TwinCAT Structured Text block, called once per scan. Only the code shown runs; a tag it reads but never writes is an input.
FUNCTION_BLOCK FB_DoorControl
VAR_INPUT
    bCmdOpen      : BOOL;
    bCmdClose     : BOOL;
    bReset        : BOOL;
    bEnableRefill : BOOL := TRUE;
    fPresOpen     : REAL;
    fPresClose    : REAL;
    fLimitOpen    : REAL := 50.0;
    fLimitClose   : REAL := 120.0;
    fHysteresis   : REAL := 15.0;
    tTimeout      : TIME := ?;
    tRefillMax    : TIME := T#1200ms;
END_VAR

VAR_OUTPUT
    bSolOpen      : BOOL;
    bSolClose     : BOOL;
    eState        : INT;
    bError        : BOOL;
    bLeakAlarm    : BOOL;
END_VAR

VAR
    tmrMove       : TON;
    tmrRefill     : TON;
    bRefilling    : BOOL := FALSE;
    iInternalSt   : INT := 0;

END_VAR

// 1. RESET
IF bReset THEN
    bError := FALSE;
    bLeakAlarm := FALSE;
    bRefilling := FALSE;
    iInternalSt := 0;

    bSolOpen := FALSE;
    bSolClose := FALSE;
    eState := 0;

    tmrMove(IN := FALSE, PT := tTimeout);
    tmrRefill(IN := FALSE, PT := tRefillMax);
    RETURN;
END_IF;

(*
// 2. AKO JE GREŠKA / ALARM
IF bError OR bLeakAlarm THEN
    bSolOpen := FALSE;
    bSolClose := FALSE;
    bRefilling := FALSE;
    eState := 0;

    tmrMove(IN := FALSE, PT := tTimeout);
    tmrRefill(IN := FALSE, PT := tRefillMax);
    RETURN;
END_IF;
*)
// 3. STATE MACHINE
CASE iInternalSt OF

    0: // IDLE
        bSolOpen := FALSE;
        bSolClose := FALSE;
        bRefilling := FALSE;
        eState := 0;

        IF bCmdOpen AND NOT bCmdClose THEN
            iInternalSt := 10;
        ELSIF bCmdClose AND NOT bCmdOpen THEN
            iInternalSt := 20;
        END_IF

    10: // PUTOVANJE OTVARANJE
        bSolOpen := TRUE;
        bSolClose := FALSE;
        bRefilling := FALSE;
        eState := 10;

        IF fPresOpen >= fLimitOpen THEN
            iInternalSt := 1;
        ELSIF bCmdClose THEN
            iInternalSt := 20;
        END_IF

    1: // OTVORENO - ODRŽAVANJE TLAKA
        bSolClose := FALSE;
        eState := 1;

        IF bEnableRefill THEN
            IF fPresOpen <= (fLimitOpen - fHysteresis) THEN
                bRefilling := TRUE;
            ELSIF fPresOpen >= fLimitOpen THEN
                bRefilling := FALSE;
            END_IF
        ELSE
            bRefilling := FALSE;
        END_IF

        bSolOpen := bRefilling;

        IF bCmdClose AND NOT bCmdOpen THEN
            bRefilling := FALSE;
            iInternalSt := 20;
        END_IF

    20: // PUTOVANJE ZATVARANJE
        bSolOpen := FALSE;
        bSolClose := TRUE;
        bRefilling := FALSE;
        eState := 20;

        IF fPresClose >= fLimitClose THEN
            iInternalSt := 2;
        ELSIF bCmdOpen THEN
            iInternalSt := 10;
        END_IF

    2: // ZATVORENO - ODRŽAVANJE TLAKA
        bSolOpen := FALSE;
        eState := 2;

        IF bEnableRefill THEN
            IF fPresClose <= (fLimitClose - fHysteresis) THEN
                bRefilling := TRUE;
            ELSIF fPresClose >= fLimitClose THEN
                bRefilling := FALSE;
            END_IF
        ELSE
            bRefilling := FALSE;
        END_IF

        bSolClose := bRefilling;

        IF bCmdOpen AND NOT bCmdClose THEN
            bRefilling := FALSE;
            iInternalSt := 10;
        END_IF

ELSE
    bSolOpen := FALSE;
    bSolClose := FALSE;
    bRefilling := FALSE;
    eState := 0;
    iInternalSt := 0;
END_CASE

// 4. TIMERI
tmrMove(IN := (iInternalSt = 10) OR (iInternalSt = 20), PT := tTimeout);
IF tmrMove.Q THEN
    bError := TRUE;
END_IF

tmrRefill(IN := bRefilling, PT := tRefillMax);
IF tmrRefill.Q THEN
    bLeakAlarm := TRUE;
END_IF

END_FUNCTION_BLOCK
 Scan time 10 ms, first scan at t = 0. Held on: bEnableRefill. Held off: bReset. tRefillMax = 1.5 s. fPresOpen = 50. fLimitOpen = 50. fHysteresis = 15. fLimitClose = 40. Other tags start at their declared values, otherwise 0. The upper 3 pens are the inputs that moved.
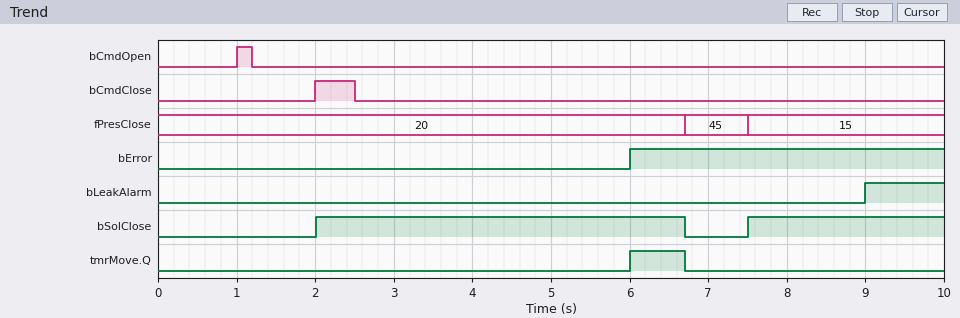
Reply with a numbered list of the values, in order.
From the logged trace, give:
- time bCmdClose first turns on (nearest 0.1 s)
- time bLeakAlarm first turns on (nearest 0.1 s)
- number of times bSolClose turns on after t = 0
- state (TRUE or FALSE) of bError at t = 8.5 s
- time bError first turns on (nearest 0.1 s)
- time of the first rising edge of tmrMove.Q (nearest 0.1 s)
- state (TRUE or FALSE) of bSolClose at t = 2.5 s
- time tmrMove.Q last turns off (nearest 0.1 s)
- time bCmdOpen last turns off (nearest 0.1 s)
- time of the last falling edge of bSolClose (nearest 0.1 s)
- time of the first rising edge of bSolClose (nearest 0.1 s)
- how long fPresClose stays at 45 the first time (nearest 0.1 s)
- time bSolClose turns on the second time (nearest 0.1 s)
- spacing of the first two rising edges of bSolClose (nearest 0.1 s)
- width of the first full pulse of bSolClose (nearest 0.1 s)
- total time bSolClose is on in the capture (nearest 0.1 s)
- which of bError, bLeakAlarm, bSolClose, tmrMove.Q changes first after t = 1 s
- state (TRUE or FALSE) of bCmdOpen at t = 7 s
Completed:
1. 2.0 s
2. 9.0 s
3. 2
4. TRUE
5. 6.0 s
6. 6.0 s
7. TRUE
8. 6.7 s
9. 1.2 s
10. 6.7 s
11. 2.0 s
12. 0.8 s
13. 7.5 s
14. 5.5 s
15. 4.7 s
16. 7.2 s
17. bSolClose
18. FALSE
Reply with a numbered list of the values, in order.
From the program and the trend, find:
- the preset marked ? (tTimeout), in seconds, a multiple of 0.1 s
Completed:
1. 4.0 s
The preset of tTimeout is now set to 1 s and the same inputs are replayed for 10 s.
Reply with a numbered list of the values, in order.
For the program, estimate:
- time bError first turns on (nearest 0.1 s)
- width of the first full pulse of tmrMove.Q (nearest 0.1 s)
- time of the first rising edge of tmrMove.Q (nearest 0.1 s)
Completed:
1. 3.0 s
2. 3.7 s
3. 3.0 s
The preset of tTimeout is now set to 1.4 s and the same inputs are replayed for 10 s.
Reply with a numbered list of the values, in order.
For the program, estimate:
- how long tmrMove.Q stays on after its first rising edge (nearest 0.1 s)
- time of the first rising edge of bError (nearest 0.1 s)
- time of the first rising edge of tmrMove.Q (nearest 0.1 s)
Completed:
1. 3.3 s
2. 3.4 s
3. 3.4 s
